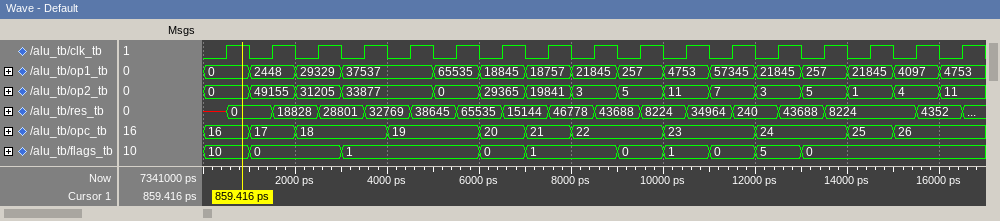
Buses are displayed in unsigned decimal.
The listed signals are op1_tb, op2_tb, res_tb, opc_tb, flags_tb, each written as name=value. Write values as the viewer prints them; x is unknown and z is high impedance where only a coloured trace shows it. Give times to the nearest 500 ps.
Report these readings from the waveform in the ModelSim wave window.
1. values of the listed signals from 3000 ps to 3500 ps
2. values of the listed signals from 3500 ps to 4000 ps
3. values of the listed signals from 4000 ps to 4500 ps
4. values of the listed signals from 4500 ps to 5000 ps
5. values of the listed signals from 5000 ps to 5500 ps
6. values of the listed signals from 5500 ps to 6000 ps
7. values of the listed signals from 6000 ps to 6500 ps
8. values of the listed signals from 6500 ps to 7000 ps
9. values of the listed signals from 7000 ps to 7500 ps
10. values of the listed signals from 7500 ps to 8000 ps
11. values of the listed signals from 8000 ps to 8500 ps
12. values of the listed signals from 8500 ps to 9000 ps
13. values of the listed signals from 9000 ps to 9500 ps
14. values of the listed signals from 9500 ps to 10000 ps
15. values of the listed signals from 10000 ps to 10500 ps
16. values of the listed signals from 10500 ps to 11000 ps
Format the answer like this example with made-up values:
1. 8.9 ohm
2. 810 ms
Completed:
1. op1_tb=37537, op2_tb=33877, res_tb=28801, opc_tb=18, flags_tb=1
2. op1_tb=37537, op2_tb=33877, res_tb=32769, opc_tb=18, flags_tb=1
3. op1_tb=37537, op2_tb=33877, res_tb=32769, opc_tb=19, flags_tb=1
4. op1_tb=37537, op2_tb=33877, res_tb=38645, opc_tb=19, flags_tb=1
5. op1_tb=65535, op2_tb=0, res_tb=38645, opc_tb=19, flags_tb=1
6. op1_tb=65535, op2_tb=0, res_tb=65535, opc_tb=19, flags_tb=1
7. op1_tb=18845, op2_tb=29365, res_tb=65535, opc_tb=20, flags_tb=0
8. op1_tb=18845, op2_tb=29365, res_tb=15144, opc_tb=20, flags_tb=0
9. op1_tb=18757, op2_tb=19841, res_tb=15144, opc_tb=21, flags_tb=1
10. op1_tb=18757, op2_tb=19841, res_tb=46778, opc_tb=21, flags_tb=1
11. op1_tb=21845, op2_tb=3, res_tb=46778, opc_tb=22, flags_tb=1
12. op1_tb=21845, op2_tb=3, res_tb=43688, opc_tb=22, flags_tb=1
13. op1_tb=257, op2_tb=5, res_tb=43688, opc_tb=22, flags_tb=0
14. op1_tb=257, op2_tb=5, res_tb=8224, opc_tb=22, flags_tb=0
15. op1_tb=4753, op2_tb=11, res_tb=8224, opc_tb=23, flags_tb=1
16. op1_tb=4753, op2_tb=11, res_tb=34964, opc_tb=23, flags_tb=1
